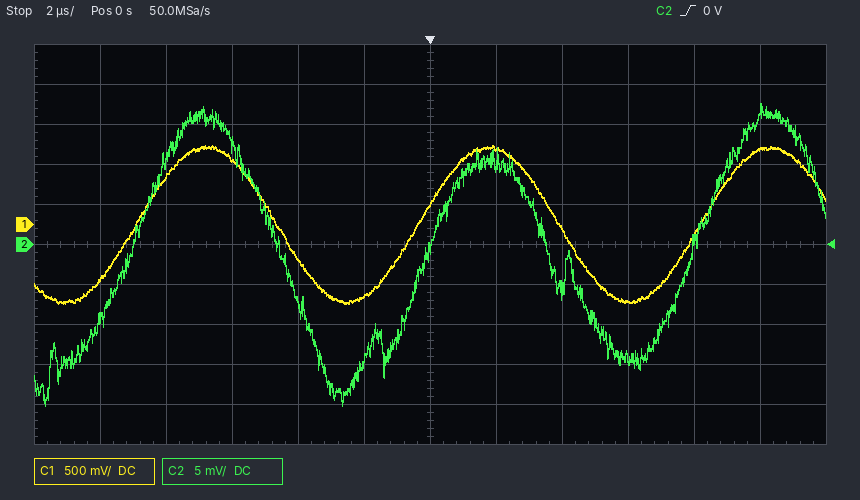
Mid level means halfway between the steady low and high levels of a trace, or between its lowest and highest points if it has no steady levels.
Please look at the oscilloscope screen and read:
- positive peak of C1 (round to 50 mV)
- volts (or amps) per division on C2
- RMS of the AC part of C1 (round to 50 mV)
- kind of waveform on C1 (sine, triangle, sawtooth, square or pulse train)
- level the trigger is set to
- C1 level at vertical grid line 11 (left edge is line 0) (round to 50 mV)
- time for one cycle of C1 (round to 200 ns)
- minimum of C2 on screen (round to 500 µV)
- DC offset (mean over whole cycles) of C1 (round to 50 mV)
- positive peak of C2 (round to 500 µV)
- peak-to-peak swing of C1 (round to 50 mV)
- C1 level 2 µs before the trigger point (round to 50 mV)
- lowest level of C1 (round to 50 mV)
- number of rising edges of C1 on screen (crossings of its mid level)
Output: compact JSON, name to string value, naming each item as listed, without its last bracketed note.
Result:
{"positive peak of C1": "1.00 V", "volts (or amps) per division on C2": "5 mV", "RMS of the AC part of C1": "700 mV", "kind of waveform on C1": "sine", "level the trigger is set to": "0 V", "C1 level at vertical grid line 11 (left edge is line 0)": "950 mV", "time for one cycle of C1": "8.6 µs", "minimum of C2 on screen": "-20.0 mV", "DC offset (mean over whole cycles) of C1": "0 mV", "positive peak of C2": "17.5 mV", "peak-to-peak swing of C1": "2.00 V", "C1 level 2 µs before the trigger point": "-900 mV", "lowest level of C1": "-1.00 V", "number of rising edges of C1 on screen": "3"}
